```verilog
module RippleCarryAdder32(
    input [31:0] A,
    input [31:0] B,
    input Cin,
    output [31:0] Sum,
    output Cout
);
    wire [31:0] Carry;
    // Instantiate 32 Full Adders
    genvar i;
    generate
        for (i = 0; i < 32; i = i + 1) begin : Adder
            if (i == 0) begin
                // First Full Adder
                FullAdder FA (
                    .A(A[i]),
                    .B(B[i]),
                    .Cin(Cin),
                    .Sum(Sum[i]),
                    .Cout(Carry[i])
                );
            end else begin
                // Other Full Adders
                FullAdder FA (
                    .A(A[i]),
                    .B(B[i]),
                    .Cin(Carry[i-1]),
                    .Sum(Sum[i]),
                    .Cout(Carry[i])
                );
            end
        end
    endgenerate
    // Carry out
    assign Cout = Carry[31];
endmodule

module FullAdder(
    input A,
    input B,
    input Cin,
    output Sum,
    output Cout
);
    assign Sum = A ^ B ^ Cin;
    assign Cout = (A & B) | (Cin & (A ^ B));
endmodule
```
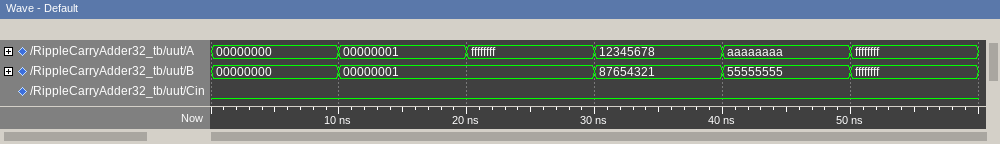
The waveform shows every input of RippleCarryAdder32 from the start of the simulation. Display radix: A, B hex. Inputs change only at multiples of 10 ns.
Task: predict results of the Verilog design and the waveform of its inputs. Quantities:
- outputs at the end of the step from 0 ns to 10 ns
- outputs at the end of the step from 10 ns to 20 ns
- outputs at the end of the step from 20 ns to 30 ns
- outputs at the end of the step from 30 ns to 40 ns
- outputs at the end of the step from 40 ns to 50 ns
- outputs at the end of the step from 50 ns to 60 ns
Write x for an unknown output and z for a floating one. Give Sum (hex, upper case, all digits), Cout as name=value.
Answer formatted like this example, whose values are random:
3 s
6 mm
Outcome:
Sum=00000000, Cout=0
Sum=00000002, Cout=0
Sum=00000000, Cout=1
Sum=99999999, Cout=0
Sum=FFFFFFFF, Cout=0
Sum=FFFFFFFE, Cout=1
